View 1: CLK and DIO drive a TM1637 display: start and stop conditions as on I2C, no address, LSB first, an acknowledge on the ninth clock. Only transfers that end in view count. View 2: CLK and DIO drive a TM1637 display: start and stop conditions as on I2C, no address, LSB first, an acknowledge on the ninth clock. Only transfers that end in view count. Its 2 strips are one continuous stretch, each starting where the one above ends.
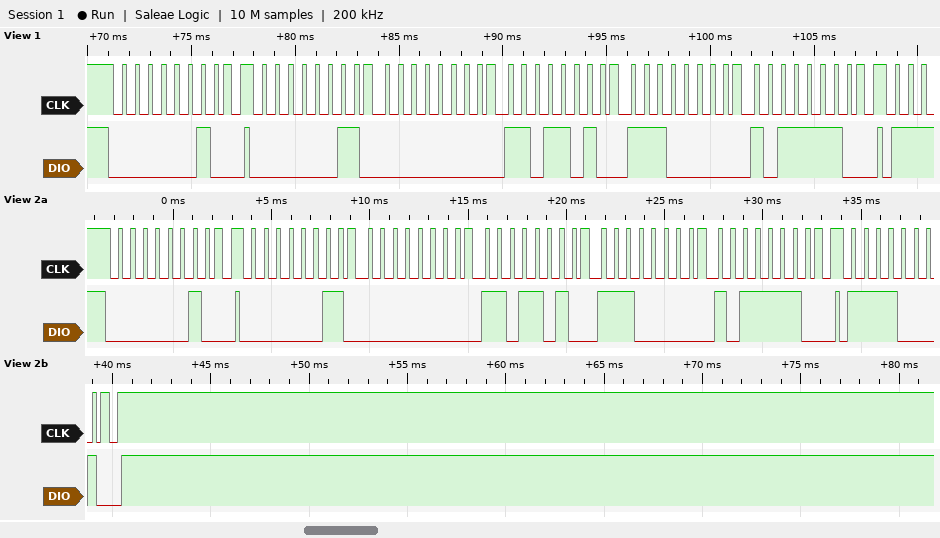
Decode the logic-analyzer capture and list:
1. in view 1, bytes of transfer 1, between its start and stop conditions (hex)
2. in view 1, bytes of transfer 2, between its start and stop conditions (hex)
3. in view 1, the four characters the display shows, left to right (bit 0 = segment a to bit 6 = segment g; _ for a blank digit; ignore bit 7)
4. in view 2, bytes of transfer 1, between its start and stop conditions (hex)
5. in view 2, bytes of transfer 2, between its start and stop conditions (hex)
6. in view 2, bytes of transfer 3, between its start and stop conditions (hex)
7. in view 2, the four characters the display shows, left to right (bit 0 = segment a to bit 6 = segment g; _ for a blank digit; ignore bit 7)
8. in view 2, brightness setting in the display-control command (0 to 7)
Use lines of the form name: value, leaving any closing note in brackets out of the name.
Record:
in view 1, bytes of transfer 1, between its start and stop conditions: 40
in view 1, bytes of transfer 2, between its start and stop conditions: C0 00 5B 07 7D
in view 1, the four characters the display shows, left to right: _276
in view 2, bytes of transfer 1, between its start and stop conditions: 40
in view 2, bytes of transfer 2, between its start and stop conditions: C0 00 5B 07 7D
in view 2, bytes of transfer 3, between its start and stop conditions: 8F
in view 2, the four characters the display shows, left to right: _276
in view 2, brightness setting in the display-control command: 7
